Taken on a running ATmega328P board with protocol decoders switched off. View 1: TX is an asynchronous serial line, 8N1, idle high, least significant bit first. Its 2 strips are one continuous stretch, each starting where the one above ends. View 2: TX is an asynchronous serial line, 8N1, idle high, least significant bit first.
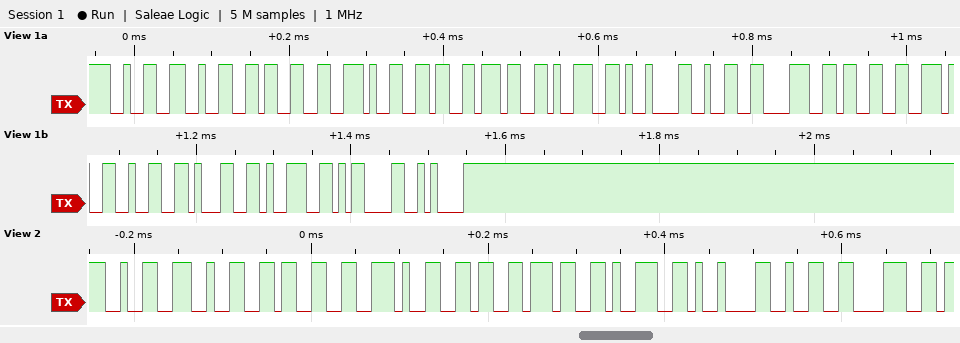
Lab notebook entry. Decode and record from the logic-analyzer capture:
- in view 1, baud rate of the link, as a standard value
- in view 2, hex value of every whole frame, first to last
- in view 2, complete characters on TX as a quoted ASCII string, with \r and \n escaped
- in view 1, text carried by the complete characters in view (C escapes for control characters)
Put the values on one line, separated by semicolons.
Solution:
115200 baud; 0x32 0x32 0x33 0x2E 0x36 0x37 0x39 0x09 0x32 0x38; "223.679\t28"; "223.679\t283.219\r\n"
